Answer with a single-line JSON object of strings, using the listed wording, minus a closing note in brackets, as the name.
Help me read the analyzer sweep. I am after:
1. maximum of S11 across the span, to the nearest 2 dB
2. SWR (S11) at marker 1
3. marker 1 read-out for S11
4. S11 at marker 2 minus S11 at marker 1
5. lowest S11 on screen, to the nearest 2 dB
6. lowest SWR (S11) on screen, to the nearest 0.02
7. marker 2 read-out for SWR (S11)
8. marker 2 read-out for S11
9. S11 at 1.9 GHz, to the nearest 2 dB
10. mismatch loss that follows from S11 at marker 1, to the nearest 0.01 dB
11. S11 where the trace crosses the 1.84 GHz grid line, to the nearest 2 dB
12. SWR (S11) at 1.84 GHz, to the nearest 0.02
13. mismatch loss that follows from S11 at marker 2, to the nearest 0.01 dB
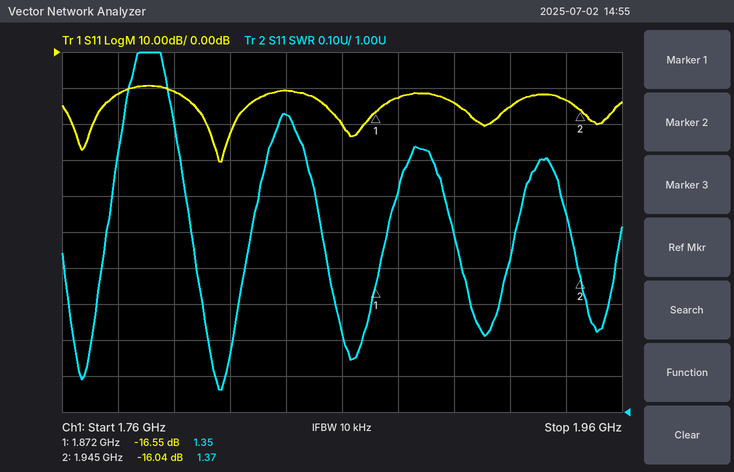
{"maximum of S11 across the span, to the nearest 2 dB": "-10 dB", "SWR (S11) at marker 1": "1.35", "marker 1 read-out for S11": "-16.55 dB", "S11 at marker 2 minus S11 at marker 1": "0.51 dB", "lowest S11 on screen, to the nearest 2 dB": "-30 dB", "lowest SWR (S11) on screen, to the nearest 0.02": "1.06", "marker 2 read-out for SWR": "1.37", "marker 2 read-out for S11": "-16.04 dB", "S11 at 1.9 GHz, to the nearest 2 dB": "-14 dB", "mismatch loss that follows from S11 at marker 1, to the nearest 0.01 dB": "0.10 dB", "S11 where the trace crosses the 1.84 GHz grid line, to the nearest 2 dB": "-10 dB", "SWR (S11) at 1.84 GHz, to the nearest 0.02": "1.82", "mismatch loss that follows from S11 at marker 2, to the nearest 0.01 dB": "0.11 dB"}
